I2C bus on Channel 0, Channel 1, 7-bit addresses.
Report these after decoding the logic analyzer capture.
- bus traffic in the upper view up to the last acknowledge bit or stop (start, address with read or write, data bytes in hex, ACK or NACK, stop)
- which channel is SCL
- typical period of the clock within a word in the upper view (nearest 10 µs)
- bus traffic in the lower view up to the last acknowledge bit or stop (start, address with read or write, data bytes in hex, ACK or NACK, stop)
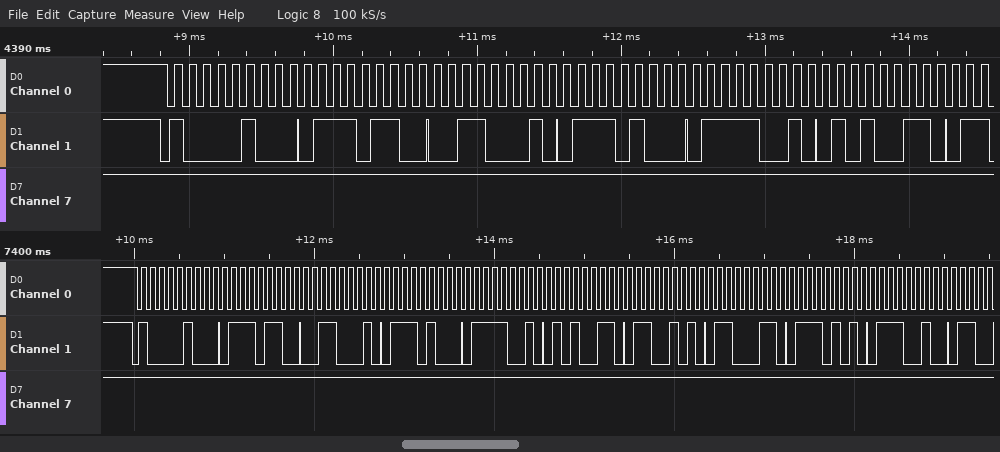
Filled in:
start, address 42 write ACK, 76 ACK, 31 ACK, 74 ACK, 79 ACK, 53 ACK
Channel 0
100 µs
start, address 42 write ACK, 76 ACK, 31 ACK, 74 ACK, 79 ACK, 53 ACK, 65 ACK, 63 ACK, 75 ACK, 72 ACK
